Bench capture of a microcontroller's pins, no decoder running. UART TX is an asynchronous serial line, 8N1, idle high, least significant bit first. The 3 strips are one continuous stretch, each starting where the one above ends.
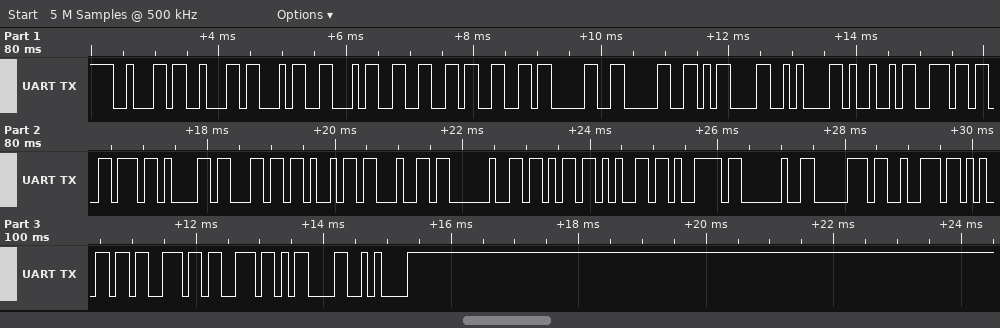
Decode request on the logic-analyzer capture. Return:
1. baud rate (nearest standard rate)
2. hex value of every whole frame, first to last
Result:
9600 baud
62 62 34 34 66 66 30 30 0D 0A 49 6E 76 61 6C 69 64 20 6B 65 79 20 70 72 65 73 73 0D 0A
